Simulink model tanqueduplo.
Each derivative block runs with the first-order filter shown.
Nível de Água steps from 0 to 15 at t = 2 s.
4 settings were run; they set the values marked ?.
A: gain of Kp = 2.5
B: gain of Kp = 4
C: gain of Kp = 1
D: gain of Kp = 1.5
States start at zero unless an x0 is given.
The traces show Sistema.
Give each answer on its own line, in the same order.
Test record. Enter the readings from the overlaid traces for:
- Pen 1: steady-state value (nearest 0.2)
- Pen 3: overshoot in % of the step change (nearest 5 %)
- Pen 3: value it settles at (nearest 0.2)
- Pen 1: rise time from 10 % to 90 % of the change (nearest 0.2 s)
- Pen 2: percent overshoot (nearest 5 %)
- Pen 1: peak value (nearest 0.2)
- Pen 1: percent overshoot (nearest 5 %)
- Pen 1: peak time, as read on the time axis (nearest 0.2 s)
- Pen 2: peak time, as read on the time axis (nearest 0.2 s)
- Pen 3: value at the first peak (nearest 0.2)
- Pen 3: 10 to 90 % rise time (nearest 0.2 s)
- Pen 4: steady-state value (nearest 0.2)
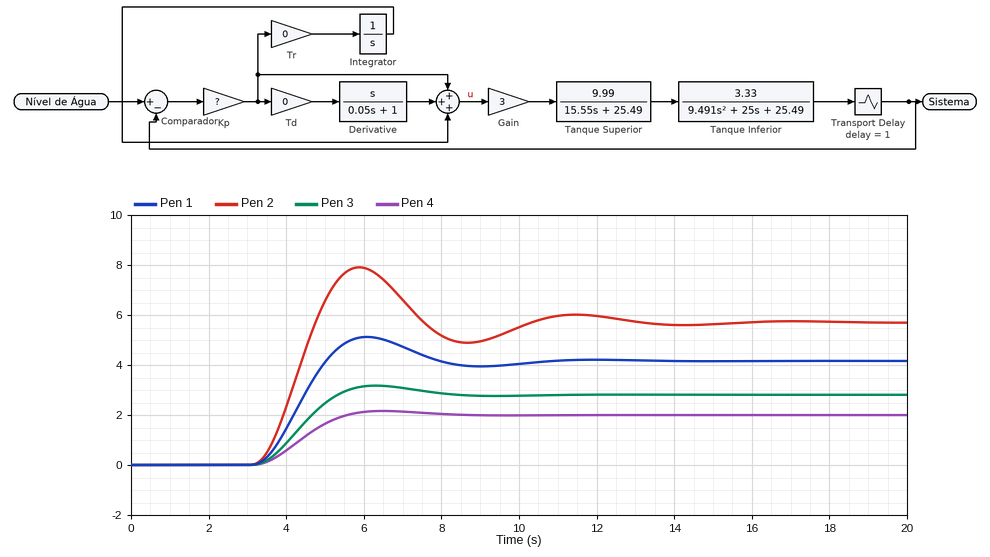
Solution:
4.2
15 %
2.8
1.2 s
40 %
5.2
25 %
6.0 s
5.8 s
3.2
1.4 s
2.0
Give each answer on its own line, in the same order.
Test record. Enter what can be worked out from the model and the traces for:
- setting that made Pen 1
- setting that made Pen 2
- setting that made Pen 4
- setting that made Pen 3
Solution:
A
B
C
D
